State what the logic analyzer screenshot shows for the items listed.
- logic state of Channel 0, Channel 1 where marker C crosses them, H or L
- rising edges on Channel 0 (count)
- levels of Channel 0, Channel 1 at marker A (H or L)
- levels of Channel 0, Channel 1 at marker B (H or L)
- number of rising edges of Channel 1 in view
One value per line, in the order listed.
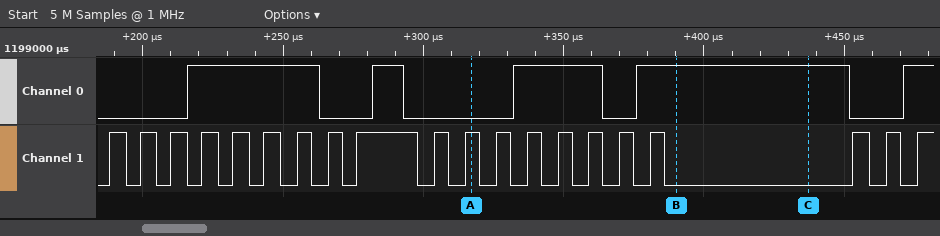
Channel 0=H, Channel 1=L
5
Channel 0=L, Channel 1=H
Channel 0=H, Channel 1=L
20
